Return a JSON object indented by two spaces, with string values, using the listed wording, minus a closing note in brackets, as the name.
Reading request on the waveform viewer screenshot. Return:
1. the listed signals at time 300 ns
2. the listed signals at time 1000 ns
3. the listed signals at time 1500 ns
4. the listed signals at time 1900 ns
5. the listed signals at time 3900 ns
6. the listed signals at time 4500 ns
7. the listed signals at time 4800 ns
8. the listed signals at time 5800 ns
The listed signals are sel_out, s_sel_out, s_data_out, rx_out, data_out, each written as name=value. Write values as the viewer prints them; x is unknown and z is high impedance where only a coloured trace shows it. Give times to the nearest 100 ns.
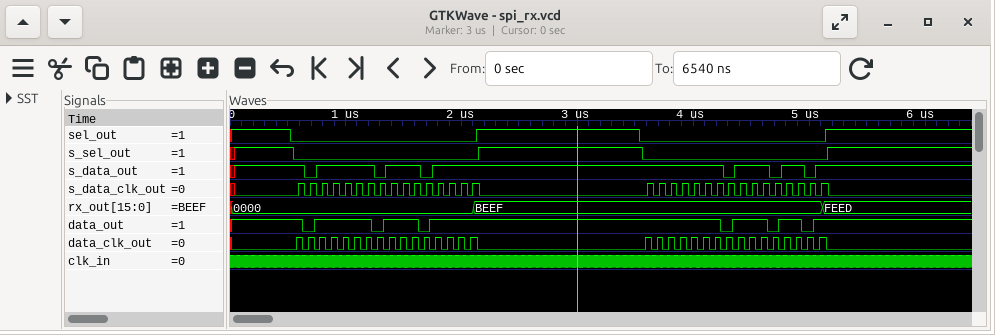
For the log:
{
  "the listed signals at time 300 ns": "sel_out=1, s_sel_out=1, s_data_out=1, rx_out=0000, data_out=1",
  "the listed signals at time 1000 ns": "sel_out=0, s_sel_out=0, s_data_out=1, rx_out=0000, data_out=1",
  "the listed signals at time 1500 ns": "sel_out=0, s_sel_out=0, s_data_out=1, rx_out=0000, data_out=1",
  "the listed signals at time 1900 ns": "sel_out=0, s_sel_out=0, s_data_out=1, rx_out=0000, data_out=1",
  "the listed signals at time 3900 ns": "sel_out=0, s_sel_out=0, s_data_out=1, rx_out=BEEF, data_out=1",
  "the listed signals at time 4500 ns": "sel_out=0, s_sel_out=0, s_data_out=1, rx_out=BEEF, data_out=1",
  "the listed signals at time 4800 ns": "sel_out=0, s_sel_out=0, s_data_out=1, rx_out=BEEF, data_out=1",
  "the listed signals at time 5800 ns": "sel_out=1, s_sel_out=1, s_data_out=1, rx_out=FEED, data_out=1"
}
